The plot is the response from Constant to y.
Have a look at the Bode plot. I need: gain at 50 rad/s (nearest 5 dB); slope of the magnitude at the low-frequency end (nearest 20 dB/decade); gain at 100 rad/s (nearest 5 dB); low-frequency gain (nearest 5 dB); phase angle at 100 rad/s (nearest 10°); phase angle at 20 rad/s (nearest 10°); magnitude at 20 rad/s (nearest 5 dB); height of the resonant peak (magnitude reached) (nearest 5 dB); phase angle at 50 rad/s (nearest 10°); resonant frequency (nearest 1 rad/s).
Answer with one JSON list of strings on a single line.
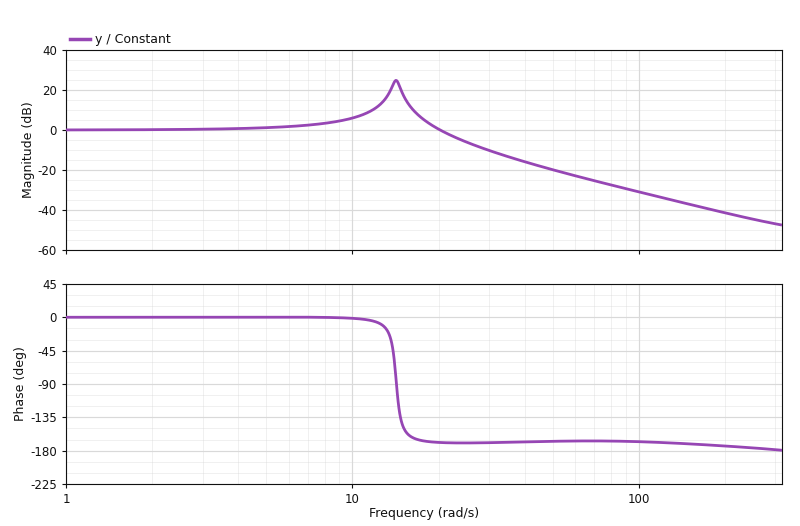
["-20 dB", "0 dB/decade", "-30 dB", "0 dB", "-170°", "-170°", "0 dB", "25 dB", "-170°", "14 rad/s"]
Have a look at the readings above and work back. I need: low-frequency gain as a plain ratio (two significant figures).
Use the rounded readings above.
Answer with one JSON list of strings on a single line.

["1.0"]
